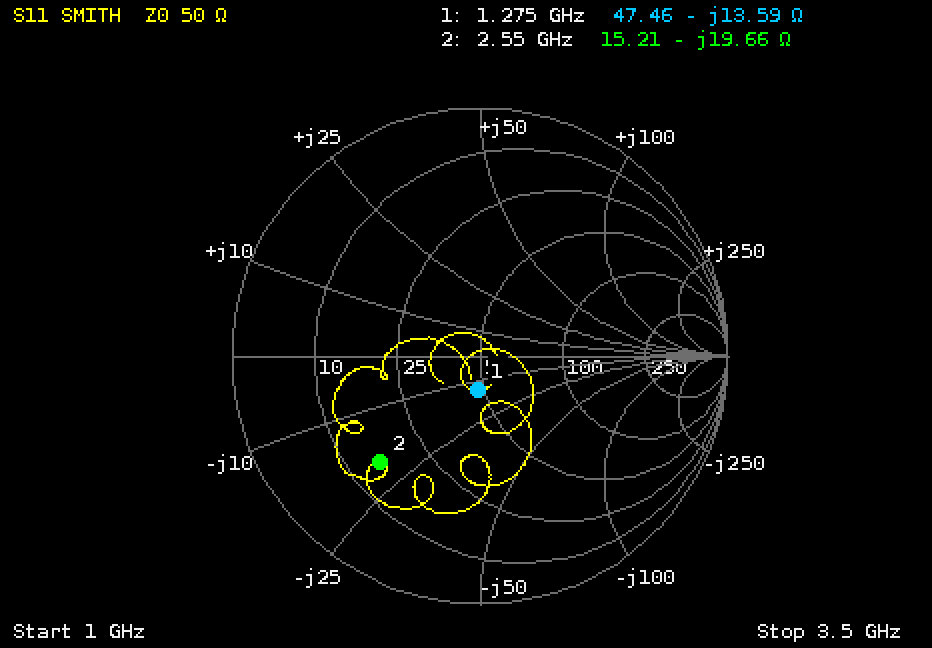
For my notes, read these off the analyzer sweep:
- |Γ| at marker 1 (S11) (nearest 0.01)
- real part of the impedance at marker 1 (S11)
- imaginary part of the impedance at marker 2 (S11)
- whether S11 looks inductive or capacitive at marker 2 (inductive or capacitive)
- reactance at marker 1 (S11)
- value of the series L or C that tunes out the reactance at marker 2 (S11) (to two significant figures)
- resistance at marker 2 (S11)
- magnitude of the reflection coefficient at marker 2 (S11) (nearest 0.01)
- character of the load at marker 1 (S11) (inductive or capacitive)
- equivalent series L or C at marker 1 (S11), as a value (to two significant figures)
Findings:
0.14
47.46 Ω
-19.66 Ω
capacitive
-13.59 Ω
1.2 nH
15.21 Ω
0.59
capacitive
9.2 pF
